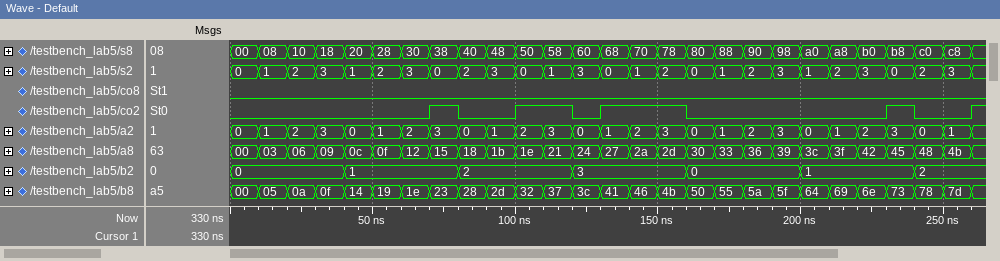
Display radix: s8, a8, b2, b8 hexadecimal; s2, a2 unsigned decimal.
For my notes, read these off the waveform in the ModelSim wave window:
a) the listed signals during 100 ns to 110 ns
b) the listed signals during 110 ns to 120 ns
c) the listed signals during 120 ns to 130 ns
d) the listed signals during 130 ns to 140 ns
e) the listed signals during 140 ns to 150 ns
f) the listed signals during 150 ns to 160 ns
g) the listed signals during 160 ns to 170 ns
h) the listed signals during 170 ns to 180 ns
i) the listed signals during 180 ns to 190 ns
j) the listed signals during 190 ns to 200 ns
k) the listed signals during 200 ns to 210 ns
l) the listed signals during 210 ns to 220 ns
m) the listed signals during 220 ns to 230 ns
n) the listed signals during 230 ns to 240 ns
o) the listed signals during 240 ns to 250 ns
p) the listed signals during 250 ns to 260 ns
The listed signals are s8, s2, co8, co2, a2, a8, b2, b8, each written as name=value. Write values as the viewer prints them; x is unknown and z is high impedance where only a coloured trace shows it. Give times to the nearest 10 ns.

s8=50, s2=0, co8=0, co2=1, a2=2, a8=1e, b2=2, b8=32
s8=58, s2=1, co8=0, co2=1, a2=3, a8=21, b2=2, b8=37
s8=60, s2=3, co8=0, co2=0, a2=0, a8=24, b2=3, b8=3c
s8=68, s2=0, co8=0, co2=1, a2=1, a8=27, b2=3, b8=41
s8=70, s2=1, co8=0, co2=1, a2=2, a8=2a, b2=3, b8=46
s8=78, s2=2, co8=0, co2=1, a2=3, a8=2d, b2=3, b8=4b
s8=80, s2=0, co8=0, co2=0, a2=0, a8=30, b2=0, b8=50
s8=88, s2=1, co8=0, co2=0, a2=1, a8=33, b2=0, b8=55
s8=90, s2=2, co8=0, co2=0, a2=2, a8=36, b2=0, b8=5a
s8=98, s2=3, co8=0, co2=0, a2=3, a8=39, b2=0, b8=5f
s8=a0, s2=1, co8=0, co2=0, a2=0, a8=3c, b2=1, b8=64
s8=a8, s2=2, co8=0, co2=0, a2=1, a8=3f, b2=1, b8=69
s8=b0, s2=3, co8=0, co2=0, a2=2, a8=42, b2=1, b8=6e
s8=b8, s2=0, co8=0, co2=1, a2=3, a8=45, b2=1, b8=73
s8=c0, s2=2, co8=0, co2=0, a2=0, a8=48, b2=2, b8=78
s8=c8, s2=3, co8=0, co2=0, a2=1, a8=4b, b2=2, b8=7d
